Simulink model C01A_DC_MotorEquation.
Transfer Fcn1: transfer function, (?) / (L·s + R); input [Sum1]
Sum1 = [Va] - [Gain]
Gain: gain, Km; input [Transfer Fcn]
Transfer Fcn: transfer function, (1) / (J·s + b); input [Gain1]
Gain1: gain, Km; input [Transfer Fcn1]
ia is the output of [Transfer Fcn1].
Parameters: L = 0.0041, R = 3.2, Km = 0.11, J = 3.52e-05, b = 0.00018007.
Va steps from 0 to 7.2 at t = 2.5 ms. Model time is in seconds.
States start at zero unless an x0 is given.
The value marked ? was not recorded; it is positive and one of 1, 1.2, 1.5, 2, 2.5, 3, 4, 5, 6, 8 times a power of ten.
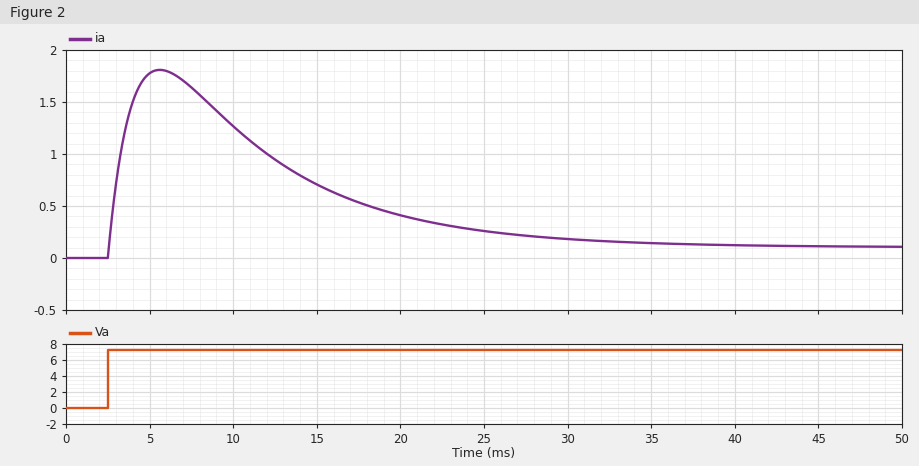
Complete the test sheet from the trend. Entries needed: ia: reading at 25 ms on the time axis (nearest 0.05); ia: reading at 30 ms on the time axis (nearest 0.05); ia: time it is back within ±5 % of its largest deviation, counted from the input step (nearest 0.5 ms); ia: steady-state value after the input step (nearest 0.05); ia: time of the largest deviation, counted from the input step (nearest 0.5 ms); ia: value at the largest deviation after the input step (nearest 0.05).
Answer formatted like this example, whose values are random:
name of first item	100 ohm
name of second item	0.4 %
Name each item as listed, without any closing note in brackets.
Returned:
ia: reading at 25 ms on the time axis	0.25
ia: reading at 30 ms on the time axis	0.20
ia: time it is back within ±5 % of its largest deviation, counted from the input step	26.5 ms
ia: steady-state value after the input step	0.10
ia: time of the largest deviation, counted from the input step	3.0 ms
ia: value at the largest deviation after the input step	1.80
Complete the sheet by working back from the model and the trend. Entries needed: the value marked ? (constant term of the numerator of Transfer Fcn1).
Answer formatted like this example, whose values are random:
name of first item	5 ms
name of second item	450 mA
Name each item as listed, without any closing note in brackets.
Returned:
the value marked ?	1
